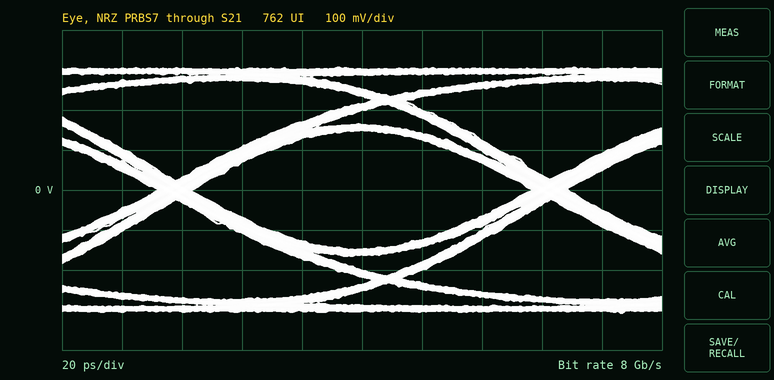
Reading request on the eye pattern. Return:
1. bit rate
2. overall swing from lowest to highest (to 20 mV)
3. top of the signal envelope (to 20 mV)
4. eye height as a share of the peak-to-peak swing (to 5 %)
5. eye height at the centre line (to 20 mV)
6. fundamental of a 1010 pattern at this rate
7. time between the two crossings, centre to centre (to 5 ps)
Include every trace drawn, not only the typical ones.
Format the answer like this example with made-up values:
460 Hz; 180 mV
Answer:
8 Gb/s; 620 mV; 300 mV; 50 %; 300 mV; 4 GHz; 125 ps
